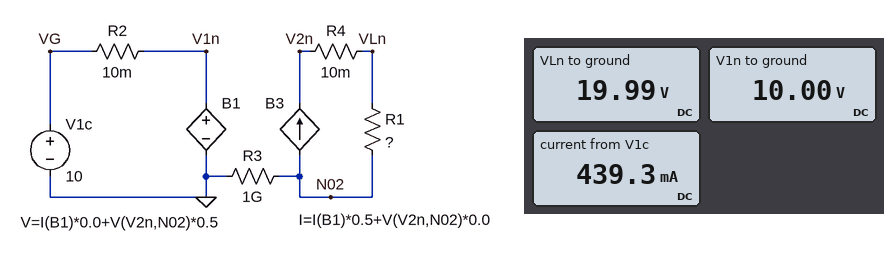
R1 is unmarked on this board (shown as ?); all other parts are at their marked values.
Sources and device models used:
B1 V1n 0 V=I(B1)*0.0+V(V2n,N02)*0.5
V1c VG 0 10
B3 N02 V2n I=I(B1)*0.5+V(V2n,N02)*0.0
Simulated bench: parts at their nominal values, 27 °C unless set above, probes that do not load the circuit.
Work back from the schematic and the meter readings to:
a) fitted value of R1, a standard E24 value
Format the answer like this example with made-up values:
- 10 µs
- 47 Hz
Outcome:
- 91 Ω
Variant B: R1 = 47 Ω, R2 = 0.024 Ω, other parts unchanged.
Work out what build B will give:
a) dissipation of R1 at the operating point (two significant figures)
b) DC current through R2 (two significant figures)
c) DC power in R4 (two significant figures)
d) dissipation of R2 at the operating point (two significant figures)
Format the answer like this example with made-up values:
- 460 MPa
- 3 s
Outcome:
- 8.5 W
- 850 mA
- 1.8 mW
- 17 mW
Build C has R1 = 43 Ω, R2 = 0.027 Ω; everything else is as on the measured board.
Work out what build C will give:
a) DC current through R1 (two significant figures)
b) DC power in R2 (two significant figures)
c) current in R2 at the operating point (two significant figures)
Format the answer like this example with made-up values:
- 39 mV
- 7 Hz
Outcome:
- 460 mA
- 23 mW
- 930 mA
